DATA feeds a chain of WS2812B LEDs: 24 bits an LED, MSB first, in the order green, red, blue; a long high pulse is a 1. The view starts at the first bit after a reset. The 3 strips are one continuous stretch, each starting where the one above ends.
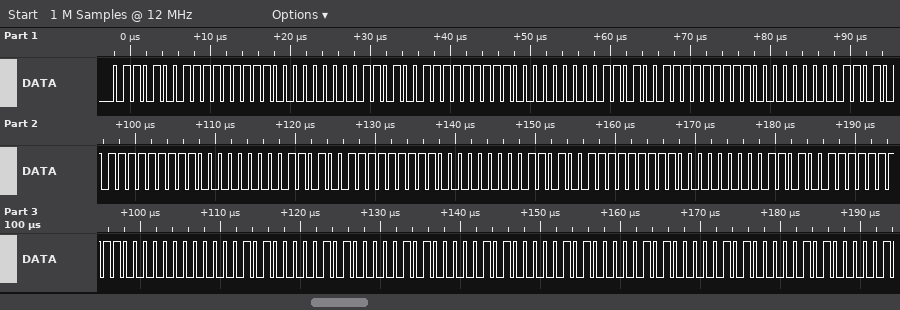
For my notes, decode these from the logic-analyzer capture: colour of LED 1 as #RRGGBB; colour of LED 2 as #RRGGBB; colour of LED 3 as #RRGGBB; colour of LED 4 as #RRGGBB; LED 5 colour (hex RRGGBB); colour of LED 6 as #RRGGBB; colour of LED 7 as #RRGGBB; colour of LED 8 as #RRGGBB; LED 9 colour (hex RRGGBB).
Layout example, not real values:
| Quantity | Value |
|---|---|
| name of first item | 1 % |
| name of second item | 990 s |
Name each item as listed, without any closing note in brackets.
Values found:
| Quantity | Value |
|---|---|
| colour of LED 1 as #RRGGBB | #FF6900 |
| colour of LED 2 as #RRGGBB | #FF6900 |
| colour of LED 3 as #RRGGBB | #FF6900 |
| colour of LED 4 as #RRGGBB | #FF6900 |
| LED 5 colour | #FF6900 |
| colour of LED 6 as #RRGGBB | #FF6900 |
| colour of LED 7 as #RRGGBB | #FF6900 |
| colour of LED 8 as #RRGGBB | #0A0A0A |
| LED 9 colour | #0A0A0A |
